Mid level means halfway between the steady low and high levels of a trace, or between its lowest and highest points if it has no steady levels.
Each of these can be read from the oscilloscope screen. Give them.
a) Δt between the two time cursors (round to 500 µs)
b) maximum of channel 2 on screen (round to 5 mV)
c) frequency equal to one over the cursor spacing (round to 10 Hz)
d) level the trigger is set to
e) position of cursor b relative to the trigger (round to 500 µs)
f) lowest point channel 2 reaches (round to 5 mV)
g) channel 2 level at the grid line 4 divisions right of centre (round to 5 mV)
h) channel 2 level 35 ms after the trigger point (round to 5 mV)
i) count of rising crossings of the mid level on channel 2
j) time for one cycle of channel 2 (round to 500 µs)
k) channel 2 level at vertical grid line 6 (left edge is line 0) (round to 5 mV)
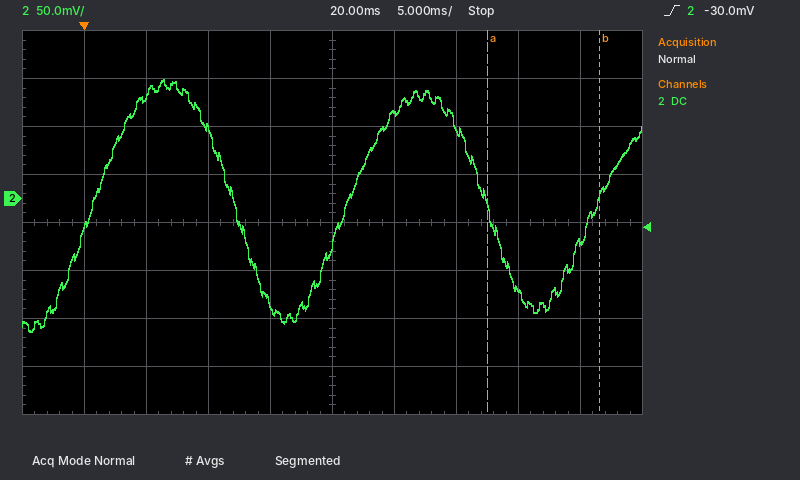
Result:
9.0 ms
125 mV
110 Hz
-30.0 mV
+41.5 ms
-140 mV
-45 mV
-95 mV
3
20.5 ms
90 mV
